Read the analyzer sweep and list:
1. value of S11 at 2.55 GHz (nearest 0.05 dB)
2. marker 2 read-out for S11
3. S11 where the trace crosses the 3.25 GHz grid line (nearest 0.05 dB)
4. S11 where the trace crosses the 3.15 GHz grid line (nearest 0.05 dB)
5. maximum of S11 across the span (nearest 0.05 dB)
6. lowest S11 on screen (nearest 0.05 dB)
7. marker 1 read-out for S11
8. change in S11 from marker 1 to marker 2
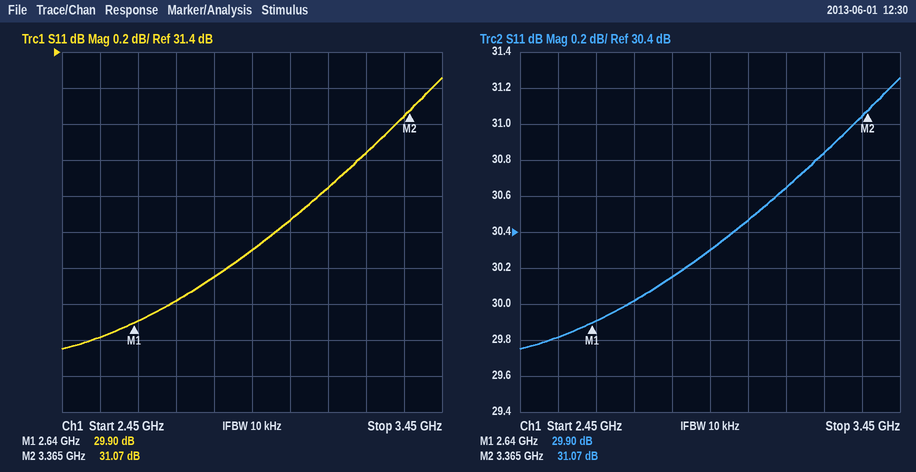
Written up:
29.80 dB
31.07 dB
30.85 dB
30.65 dB
31.25 dB
29.75 dB
29.90 dB
1.17 dB
